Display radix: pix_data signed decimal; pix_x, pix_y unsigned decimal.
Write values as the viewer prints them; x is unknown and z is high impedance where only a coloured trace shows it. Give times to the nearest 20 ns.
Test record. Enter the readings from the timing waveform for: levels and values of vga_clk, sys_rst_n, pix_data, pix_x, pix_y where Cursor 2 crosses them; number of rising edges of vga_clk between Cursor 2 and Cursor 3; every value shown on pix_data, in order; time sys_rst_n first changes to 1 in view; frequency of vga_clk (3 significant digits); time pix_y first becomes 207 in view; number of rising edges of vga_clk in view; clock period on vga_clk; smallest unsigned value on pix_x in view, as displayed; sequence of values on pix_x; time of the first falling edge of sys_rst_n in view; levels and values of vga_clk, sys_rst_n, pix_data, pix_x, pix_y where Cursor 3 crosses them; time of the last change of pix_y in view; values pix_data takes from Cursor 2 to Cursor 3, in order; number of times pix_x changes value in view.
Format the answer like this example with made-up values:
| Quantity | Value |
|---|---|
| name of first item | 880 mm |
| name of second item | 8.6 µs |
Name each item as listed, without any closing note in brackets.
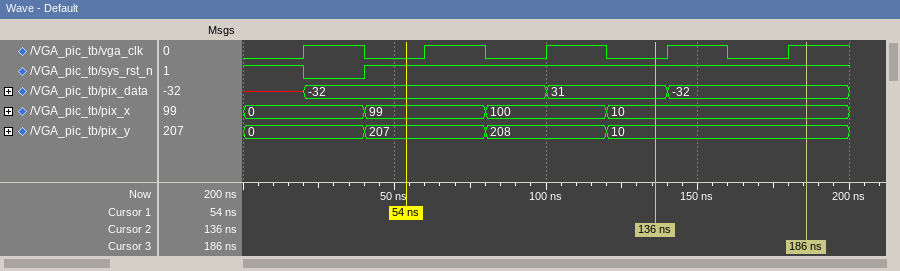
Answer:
| Quantity | Value |
|---|---|
| levels and values of vga_clk, sys_rst_n, pix_data, pix_x, pix_y where Cursor 2 crosses them | vga_clk=0, sys_rst_n=1, pix_data=31, pix_x=10, pix_y=10 |
| number of rising edges of vga_clk between Cursor 2 and Cursor 3 | 2 |
| every value shown on pix_data, in order | x, -32, 31, -32 |
| time sys_rst_n first changes to 1 in view | 40 ns |
| frequency of vga_clk | 25.0 MHz |
| time pix_y first becomes 207 in view | 40 ns |
| number of rising edges of vga_clk in view | 5 |
| clock period on vga_clk | 40 ns |
| smallest unsigned value on pix_x in view, as displayed | 0 |
| sequence of values on pix_x | 0, 99, 100, 10 |
| time of the first falling edge of sys_rst_n in view | 20 ns |
| levels and values of vga_clk, sys_rst_n, pix_data, pix_x, pix_y where Cursor 3 crosses them | vga_clk=1, sys_rst_n=1, pix_data=-32, pix_x=10, pix_y=10 |
| time of the last change of pix_y in view | 120 ns |
| values pix_data takes from Cursor 2 to Cursor 3, in order | 31, -32 |
| number of times pix_x changes value in view | 3 |
